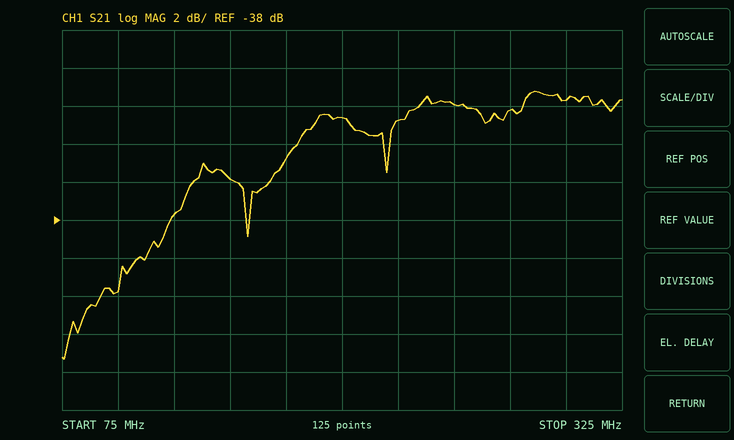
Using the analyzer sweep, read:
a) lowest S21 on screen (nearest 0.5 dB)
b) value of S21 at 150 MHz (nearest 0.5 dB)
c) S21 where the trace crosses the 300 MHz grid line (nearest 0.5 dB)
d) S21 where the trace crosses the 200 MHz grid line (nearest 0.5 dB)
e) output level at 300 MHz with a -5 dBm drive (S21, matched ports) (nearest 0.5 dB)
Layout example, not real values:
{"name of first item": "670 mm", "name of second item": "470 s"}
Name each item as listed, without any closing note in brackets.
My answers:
{"lowest S21 on screen": "-45.5 dB", "value of S21 at 150 MHz": "-36.0 dB", "S21 where the trace crosses the 300 MHz grid line": "-31.5 dB", "S21 where the trace crosses the 200 MHz grid line": "-32.5 dB", "output level at 300 MHz with a -5 dBm drive (S21, matched ports)": "-36.5 dBm"}
